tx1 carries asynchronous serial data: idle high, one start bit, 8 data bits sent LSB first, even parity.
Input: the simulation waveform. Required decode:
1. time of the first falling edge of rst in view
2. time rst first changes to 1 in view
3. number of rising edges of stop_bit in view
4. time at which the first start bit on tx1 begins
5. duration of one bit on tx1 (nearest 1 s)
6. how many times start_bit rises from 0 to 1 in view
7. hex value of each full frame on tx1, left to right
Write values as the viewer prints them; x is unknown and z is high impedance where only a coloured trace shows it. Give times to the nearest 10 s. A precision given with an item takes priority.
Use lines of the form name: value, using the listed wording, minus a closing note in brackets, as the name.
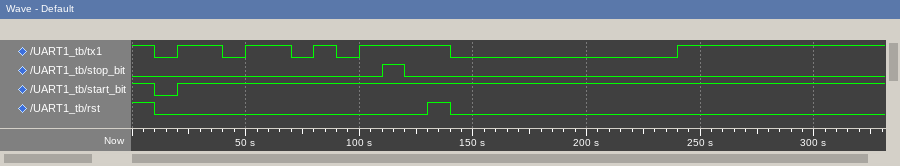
time of the first falling edge of rst in view: 10 s
time rst first changes to 1 in view: 130 s
number of rising edges of stop_bit in view: 1
time at which the first start bit on tx1 begins: 10 s
duration of one bit on tx1: 10 s
how many times start_bit rises from 0 to 1 in view: 1
hex value of each full frame on tx1, left to right: 5B, 00
